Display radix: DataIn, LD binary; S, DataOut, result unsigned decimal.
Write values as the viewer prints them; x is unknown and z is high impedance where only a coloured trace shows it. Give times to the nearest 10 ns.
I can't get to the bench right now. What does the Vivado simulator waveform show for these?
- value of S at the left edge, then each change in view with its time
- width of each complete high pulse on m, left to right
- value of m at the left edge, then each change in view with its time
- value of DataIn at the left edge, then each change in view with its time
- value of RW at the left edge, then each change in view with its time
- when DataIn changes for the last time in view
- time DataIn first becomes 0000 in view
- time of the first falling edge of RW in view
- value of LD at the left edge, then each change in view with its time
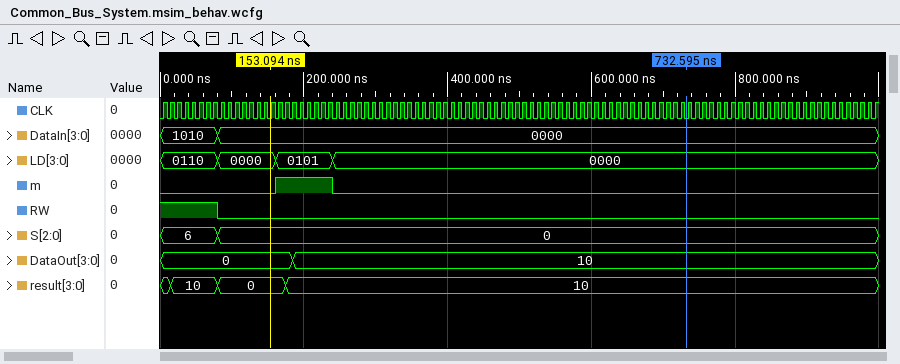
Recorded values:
6, 0 at 80 ns
80 ns
0, 1 at 160 ns, 0 at 240 ns
1010, 0000 at 80 ns
1, 0 at 80 ns
80 ns
80 ns
80 ns
0110, 0000 at 80 ns, 0101 at 160 ns, 0000 at 240 ns
